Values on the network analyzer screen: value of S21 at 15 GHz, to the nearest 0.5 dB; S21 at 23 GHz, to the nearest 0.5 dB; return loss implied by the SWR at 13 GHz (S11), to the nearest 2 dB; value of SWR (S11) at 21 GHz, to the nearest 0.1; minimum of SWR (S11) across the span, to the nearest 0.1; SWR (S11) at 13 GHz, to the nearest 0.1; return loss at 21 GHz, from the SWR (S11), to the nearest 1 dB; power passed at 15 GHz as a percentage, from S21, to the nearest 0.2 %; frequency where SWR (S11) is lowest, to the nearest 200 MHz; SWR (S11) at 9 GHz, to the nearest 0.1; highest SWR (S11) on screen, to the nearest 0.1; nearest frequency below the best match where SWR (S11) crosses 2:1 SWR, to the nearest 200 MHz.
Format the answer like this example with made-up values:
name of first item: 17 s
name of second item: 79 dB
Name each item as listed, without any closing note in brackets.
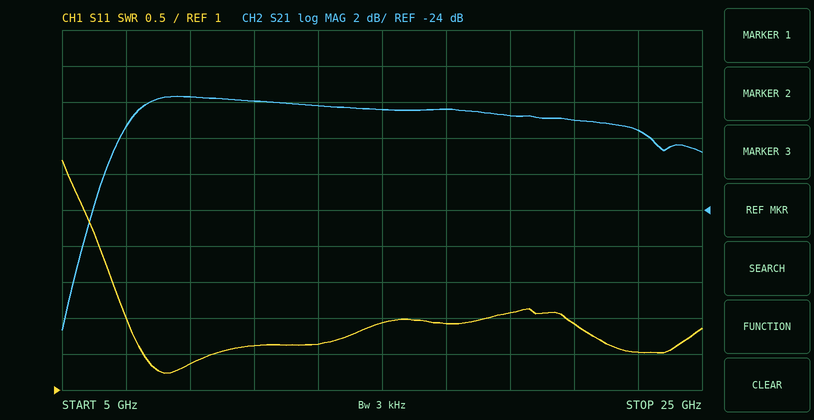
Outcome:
value of S21 at 15 GHz, to the nearest 0.5 dB: -18.5 dB
S21 at 23 GHz, to the nearest 0.5 dB: -19.5 dB
return loss implied by the SWR at 13 GHz (S11), to the nearest 2 dB: 12 dB
value of SWR (S11) at 21 GHz, to the nearest 0.1: 1.9
minimum of SWR (S11) across the span, to the nearest 0.1: 1.2
SWR (S11) at 13 GHz, to the nearest 0.1: 1.6
return loss at 21 GHz, from the SWR (S11), to the nearest 1 dB: 10 dB
power passed at 15 GHz as a percentage, from S21, to the nearest 0.2 %: 1.4 %
frequency where SWR (S11) is lowest, to the nearest 200 MHz: 8.2 GHz
SWR (S11) at 9 GHz, to the nearest 0.1: 1.4
highest SWR (S11) on screen, to the nearest 0.1: 4.2
nearest frequency below the best match where SWR (S11) crosses 2:1 SWR, to the nearest 200 MHz: 7.0 GHz
